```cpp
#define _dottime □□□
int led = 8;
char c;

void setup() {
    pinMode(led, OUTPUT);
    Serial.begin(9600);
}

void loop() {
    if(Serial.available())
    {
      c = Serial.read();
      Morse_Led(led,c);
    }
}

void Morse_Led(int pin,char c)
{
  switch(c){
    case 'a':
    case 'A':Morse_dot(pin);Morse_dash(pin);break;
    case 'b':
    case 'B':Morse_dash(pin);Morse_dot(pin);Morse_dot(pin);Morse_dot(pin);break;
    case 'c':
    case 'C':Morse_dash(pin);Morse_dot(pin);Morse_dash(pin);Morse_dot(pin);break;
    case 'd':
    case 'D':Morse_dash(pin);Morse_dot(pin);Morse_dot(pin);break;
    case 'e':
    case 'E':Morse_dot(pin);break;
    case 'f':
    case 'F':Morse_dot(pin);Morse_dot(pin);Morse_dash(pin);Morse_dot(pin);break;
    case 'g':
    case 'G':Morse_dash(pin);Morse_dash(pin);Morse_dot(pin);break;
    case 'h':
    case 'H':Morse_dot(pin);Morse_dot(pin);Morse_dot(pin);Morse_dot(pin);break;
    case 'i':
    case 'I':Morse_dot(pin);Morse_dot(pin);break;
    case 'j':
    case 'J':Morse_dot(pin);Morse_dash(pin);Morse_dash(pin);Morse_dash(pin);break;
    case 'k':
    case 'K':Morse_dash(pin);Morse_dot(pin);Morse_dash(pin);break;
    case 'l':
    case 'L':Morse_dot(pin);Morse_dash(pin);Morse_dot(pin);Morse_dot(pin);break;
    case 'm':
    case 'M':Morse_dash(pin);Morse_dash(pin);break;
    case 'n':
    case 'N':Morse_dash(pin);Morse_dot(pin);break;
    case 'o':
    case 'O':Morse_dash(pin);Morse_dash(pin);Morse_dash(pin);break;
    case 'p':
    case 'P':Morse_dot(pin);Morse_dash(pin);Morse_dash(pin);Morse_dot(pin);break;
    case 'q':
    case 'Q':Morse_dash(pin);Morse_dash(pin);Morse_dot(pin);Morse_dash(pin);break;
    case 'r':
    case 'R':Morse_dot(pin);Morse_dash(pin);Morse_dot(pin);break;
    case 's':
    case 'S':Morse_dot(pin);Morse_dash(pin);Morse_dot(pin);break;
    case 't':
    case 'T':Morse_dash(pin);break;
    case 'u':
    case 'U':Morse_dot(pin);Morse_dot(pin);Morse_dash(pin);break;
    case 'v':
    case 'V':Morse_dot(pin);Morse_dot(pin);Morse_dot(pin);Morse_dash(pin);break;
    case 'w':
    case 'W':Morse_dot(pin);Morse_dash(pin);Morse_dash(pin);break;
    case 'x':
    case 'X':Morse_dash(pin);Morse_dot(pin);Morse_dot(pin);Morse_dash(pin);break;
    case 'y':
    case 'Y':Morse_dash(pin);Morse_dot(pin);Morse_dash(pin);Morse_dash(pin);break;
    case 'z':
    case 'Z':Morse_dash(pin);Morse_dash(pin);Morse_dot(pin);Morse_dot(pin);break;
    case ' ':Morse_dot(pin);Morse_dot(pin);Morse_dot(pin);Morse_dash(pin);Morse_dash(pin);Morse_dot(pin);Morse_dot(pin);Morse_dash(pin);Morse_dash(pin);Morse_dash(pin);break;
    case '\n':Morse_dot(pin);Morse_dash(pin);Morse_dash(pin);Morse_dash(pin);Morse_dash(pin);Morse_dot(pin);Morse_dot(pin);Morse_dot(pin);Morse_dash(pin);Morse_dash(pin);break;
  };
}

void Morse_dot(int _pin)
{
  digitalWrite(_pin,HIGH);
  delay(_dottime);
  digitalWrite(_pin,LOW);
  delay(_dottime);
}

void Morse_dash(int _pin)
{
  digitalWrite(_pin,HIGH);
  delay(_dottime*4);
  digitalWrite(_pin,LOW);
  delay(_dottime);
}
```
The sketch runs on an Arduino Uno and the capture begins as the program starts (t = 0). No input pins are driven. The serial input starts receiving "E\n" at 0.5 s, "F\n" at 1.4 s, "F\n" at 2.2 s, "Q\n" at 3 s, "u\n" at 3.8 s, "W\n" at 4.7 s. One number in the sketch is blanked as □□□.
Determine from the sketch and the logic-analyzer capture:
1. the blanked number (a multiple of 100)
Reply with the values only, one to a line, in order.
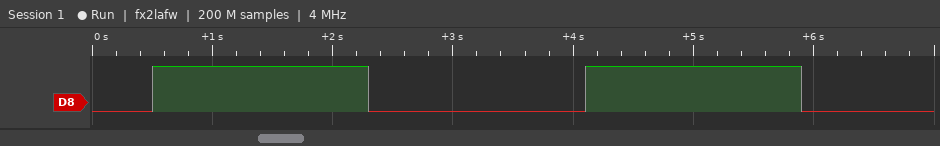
1800
